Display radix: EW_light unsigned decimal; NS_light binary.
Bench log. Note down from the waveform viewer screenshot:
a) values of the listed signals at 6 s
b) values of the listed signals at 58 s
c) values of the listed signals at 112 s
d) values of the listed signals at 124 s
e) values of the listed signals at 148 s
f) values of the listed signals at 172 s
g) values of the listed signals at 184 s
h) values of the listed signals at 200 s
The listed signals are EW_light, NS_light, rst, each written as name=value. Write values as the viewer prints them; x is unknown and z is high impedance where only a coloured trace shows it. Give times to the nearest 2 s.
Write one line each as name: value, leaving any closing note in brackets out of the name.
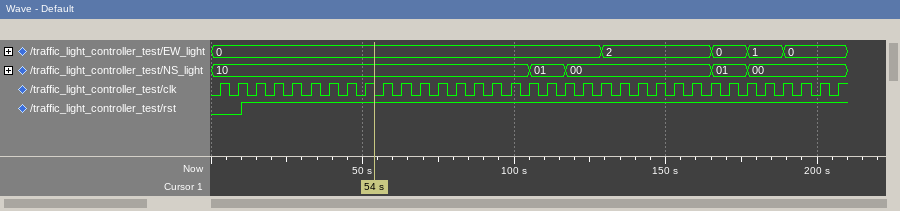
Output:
values of the listed signals at 6 s: EW_light=0, NS_light=10, rst=0
values of the listed signals at 58 s: EW_light=0, NS_light=10, rst=1
values of the listed signals at 112 s: EW_light=0, NS_light=01, rst=1
values of the listed signals at 124 s: EW_light=0, NS_light=00, rst=1
values of the listed signals at 148 s: EW_light=2, NS_light=00, rst=1
values of the listed signals at 172 s: EW_light=0, NS_light=01, rst=1
values of the listed signals at 184 s: EW_light=1, NS_light=00, rst=1
values of the listed signals at 200 s: EW_light=0, NS_light=00, rst=1
